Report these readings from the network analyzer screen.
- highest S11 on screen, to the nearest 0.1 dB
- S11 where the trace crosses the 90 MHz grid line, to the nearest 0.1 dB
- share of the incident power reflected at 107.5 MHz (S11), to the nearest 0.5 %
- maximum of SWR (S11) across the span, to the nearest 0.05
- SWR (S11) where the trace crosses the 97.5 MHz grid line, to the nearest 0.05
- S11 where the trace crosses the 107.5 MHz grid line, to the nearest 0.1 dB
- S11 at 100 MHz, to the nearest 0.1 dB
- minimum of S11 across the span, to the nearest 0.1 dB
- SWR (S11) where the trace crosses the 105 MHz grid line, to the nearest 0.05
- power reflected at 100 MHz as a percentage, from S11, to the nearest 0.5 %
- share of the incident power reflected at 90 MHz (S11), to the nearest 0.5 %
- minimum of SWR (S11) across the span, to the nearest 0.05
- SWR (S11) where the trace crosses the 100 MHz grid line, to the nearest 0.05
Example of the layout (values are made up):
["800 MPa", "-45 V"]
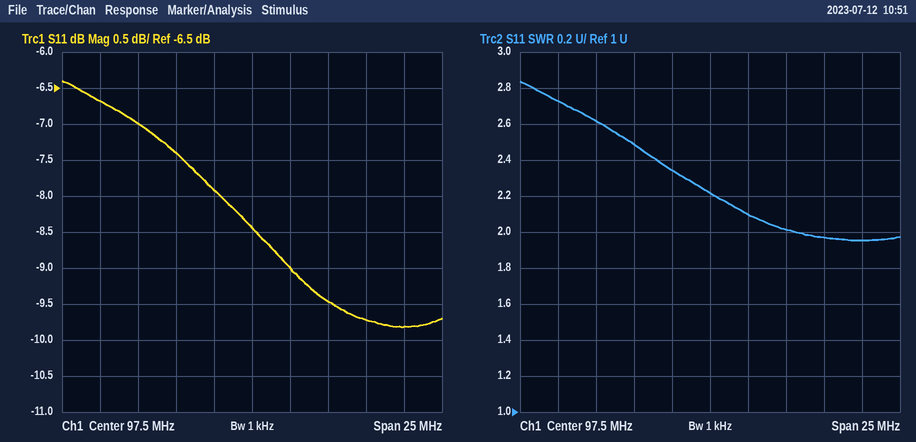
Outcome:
["-6.4 dB", "-7.0 dB", "10.5 %", "2.85", "2.20", "-9.8 dB", "-9.0 dB", "-9.8 dB", "1.95", "12.5 %", "20.0 %", "1.95", "2.10"]
